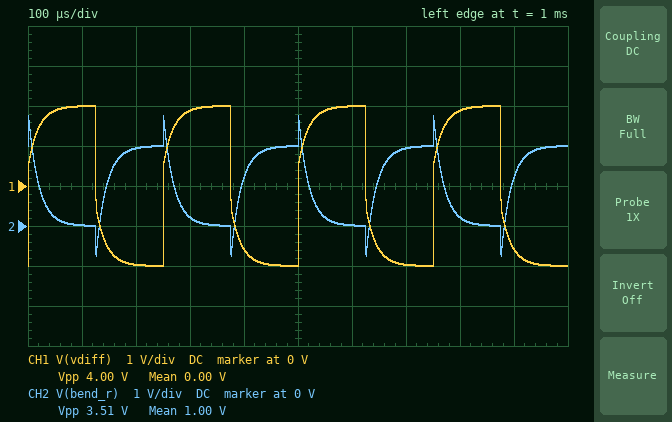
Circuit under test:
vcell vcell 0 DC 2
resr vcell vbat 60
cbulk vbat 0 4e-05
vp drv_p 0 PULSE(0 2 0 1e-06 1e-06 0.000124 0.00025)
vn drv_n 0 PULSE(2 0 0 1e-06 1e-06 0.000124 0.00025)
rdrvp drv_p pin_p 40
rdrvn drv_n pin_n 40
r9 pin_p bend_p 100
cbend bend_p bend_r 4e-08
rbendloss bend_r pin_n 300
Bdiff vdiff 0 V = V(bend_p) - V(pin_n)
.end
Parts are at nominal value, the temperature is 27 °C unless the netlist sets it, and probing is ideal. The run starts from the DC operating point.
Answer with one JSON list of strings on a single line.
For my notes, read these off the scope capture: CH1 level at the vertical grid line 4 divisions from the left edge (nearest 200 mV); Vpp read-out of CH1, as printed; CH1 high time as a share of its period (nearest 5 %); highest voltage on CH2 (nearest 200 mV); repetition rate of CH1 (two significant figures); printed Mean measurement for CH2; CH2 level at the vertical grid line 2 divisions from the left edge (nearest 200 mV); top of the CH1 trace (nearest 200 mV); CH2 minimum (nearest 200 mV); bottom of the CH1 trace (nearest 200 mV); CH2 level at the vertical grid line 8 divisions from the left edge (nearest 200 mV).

["-1.6 V", "4.00 V", "50 %", "2.8 V", "4.0 kHz", "1.00 V", "2.0 V", "2.0 V", "-800 mV", "-2.0 V", "200 mV"]
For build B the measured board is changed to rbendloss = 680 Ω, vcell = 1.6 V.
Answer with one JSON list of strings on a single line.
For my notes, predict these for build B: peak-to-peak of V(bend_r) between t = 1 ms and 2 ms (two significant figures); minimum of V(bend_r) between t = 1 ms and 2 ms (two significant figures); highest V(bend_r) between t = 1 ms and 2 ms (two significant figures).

["4.4 V", "-1.2 V", "3.2 V"]
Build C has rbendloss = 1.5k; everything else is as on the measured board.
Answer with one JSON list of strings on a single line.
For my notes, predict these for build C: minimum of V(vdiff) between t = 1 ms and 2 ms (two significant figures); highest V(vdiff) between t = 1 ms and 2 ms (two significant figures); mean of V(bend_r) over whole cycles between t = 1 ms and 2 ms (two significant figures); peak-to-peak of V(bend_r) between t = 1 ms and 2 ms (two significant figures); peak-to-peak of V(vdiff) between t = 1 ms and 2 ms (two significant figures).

["-1.9 V", "1.9 V", "1.0 V", "4.3 V", "3.9 V"]
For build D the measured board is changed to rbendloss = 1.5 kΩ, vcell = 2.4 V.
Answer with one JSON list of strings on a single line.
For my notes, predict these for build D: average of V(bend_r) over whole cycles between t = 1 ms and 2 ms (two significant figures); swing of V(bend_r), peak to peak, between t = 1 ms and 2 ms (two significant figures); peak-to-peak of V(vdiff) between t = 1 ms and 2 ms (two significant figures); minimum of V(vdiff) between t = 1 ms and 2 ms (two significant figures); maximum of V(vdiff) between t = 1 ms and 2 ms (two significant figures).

["1.0 V", "4.3 V", "3.9 V", "-1.9 V", "1.9 V"]
